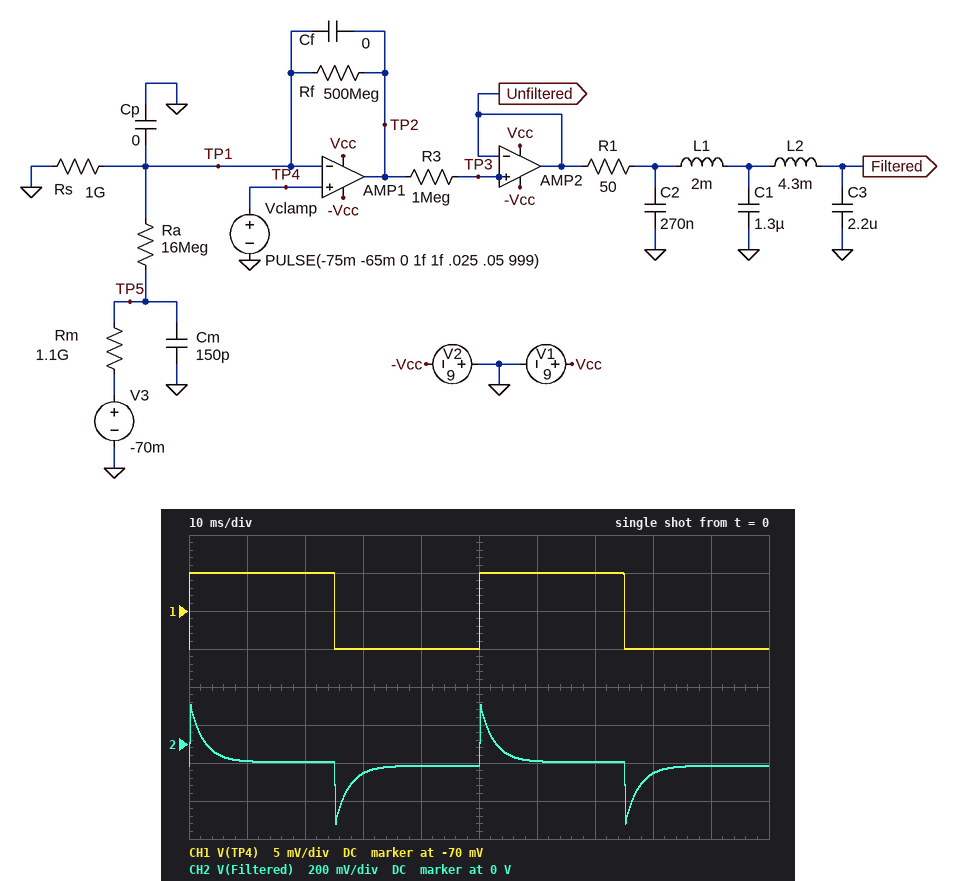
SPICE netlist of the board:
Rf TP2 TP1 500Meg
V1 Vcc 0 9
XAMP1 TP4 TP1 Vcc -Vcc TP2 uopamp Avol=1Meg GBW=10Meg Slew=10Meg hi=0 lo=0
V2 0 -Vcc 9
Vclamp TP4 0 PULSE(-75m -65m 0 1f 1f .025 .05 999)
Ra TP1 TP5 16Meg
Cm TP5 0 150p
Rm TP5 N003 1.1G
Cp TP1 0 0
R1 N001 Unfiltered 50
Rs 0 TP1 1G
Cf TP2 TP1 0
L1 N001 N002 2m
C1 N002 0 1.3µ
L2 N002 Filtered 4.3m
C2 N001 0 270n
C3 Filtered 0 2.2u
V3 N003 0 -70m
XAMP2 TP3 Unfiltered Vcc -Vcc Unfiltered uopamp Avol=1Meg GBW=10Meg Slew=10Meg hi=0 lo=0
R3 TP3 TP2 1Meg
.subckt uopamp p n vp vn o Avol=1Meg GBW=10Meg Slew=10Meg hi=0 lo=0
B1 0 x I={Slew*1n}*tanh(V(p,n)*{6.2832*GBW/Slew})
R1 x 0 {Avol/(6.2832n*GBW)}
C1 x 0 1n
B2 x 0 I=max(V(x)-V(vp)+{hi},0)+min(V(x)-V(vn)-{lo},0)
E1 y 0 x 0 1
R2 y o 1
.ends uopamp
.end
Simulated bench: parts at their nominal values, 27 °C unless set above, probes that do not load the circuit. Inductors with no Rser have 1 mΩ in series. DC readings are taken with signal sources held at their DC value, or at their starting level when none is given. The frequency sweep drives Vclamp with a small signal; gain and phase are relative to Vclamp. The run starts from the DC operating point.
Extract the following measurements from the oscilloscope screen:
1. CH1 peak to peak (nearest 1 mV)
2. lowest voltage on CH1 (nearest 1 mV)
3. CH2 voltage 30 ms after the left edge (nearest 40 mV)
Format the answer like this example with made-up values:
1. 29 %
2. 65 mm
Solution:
1. 10 mV
2. -75 mV
3. -160 mV
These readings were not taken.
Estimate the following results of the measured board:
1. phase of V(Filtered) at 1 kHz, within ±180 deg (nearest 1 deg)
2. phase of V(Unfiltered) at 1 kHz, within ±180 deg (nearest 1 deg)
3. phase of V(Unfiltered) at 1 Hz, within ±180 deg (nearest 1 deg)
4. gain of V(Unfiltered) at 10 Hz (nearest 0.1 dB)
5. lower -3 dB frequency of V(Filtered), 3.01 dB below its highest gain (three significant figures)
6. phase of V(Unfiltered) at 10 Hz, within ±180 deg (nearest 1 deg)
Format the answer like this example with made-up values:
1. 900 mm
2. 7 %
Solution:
1. -65 deg
2. 3 deg
3. 13 deg
4. 14.3 dB
5. 64.3 Hz
6. 60 deg
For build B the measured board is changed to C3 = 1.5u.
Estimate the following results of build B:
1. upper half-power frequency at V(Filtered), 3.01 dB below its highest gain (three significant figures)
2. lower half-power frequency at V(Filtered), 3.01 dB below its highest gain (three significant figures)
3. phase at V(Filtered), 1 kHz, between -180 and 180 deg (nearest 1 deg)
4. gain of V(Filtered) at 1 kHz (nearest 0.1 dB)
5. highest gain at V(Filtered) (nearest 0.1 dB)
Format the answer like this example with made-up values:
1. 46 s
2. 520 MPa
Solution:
1. 3.14 kHz
2. 70.8 Hz
3. -53 deg
4. 30.4 dB
5. 30.5 dB
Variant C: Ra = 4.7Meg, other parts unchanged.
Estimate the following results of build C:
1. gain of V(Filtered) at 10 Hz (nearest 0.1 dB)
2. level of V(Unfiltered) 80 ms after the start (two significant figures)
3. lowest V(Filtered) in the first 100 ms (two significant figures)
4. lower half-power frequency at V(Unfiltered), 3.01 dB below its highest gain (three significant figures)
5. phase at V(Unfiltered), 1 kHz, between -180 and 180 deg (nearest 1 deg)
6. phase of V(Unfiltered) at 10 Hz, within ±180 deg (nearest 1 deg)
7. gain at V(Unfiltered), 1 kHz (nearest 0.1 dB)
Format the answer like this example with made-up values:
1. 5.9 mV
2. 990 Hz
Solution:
1. 14.2 dB
2. -120 mV
3. -1.0 V
4. 226 Hz
5. 12 deg
6. 65 deg
7. 40.5 dB
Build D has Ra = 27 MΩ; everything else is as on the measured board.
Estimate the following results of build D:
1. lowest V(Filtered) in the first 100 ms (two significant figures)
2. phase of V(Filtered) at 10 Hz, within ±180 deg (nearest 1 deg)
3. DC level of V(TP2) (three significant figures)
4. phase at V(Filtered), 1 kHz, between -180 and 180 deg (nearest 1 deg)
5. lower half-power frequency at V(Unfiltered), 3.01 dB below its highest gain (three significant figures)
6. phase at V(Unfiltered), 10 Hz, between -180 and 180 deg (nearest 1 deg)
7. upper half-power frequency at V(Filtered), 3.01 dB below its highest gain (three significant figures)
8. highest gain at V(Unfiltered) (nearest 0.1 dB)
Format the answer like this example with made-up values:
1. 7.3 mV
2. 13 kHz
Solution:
1. -300 mV
2. 54 deg
3. -115 mV
4. -66 deg
5. 39.9 Hz
6. 55 deg
7. 2.31 kHz
8. 26.0 dB
